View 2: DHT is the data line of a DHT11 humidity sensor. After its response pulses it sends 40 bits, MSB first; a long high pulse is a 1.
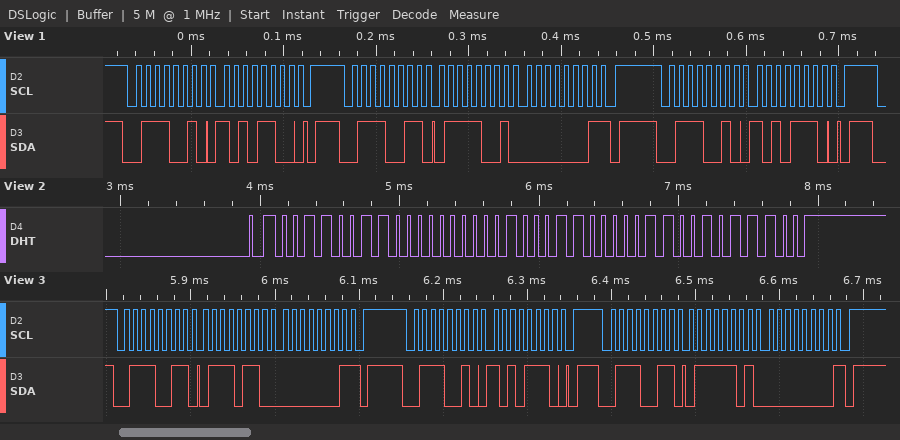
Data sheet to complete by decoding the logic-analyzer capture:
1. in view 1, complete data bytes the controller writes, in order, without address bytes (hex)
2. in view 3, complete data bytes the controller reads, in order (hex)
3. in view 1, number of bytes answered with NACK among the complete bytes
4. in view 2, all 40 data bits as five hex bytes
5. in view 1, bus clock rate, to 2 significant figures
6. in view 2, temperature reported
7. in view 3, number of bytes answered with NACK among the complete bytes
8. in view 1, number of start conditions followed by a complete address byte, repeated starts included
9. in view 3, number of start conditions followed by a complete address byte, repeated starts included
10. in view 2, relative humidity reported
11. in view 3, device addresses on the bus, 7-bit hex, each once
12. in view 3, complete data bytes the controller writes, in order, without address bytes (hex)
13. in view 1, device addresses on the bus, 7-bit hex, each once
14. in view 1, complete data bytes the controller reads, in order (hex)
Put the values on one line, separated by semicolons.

AC AE; 76 01 7D 00; 1; 33 00 23 06 5C; 100 kHz; 35.6 °C; 2; 3; 3; 51 %; 0x39; AE; 0x39; 79 01
